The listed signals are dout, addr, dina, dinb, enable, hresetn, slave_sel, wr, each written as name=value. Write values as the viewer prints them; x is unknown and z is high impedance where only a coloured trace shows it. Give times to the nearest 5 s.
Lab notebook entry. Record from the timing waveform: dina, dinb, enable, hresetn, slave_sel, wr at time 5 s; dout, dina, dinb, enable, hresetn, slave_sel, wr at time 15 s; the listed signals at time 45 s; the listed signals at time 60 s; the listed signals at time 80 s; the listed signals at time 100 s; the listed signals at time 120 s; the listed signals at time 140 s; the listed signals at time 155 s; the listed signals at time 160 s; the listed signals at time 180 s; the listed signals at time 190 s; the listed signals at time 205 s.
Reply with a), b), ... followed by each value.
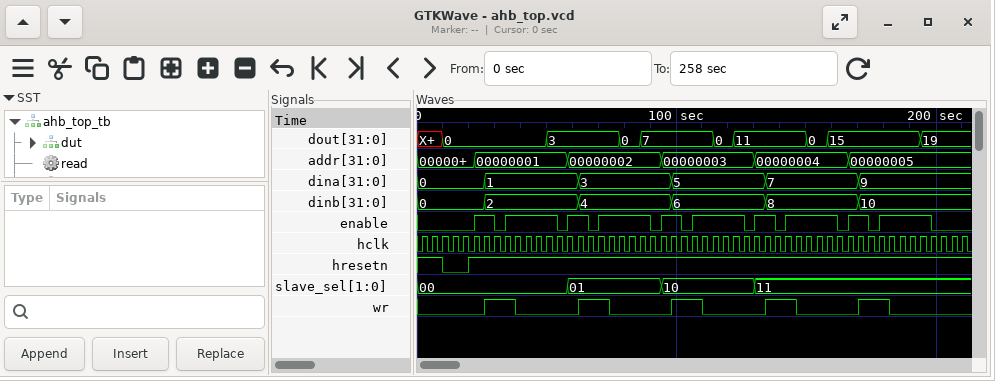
a) dina=0, dinb=0, enable=0, hresetn=1, slave_sel=00, wr=0
b) dout=0, dina=0, dinb=0, enable=0, hresetn=0, slave_sel=00, wr=0
c) dout=0, addr=00000001, dina=1, dinb=2, enable=1, hresetn=1, slave_sel=00, wr=0
d) dout=3, addr=00000002, dina=1, dinb=2, enable=1, hresetn=1, slave_sel=01, wr=0
e) dout=0, addr=00000002, dina=3, dinb=4, enable=1, hresetn=1, slave_sel=01, wr=0
f) dout=7, addr=00000003, dina=5, dinb=6, enable=1, hresetn=1, slave_sel=10, wr=1
g) dout=0, addr=00000003, dina=5, dinb=6, enable=1, hresetn=1, slave_sel=10, wr=0
h) dout=11, addr=00000004, dina=7, dinb=8, enable=0, hresetn=1, slave_sel=11, wr=1
i) dout=0, addr=00000004, dina=7, dinb=8, enable=1, hresetn=1, slave_sel=11, wr=0
j) dout=15, addr=00000004, dina=7, dinb=8, enable=1, hresetn=1, slave_sel=11, wr=0
k) dout=15, addr=00000005, dina=9, dinb=10, enable=1, hresetn=1, slave_sel=11, wr=1
l) dout=15, addr=00000005, dina=9, dinb=10, enable=1, hresetn=1, slave_sel=11, wr=0
m) dout=19, addr=00000005, dina=9, dinb=10, enable=0, hresetn=1, slave_sel=11, wr=0
